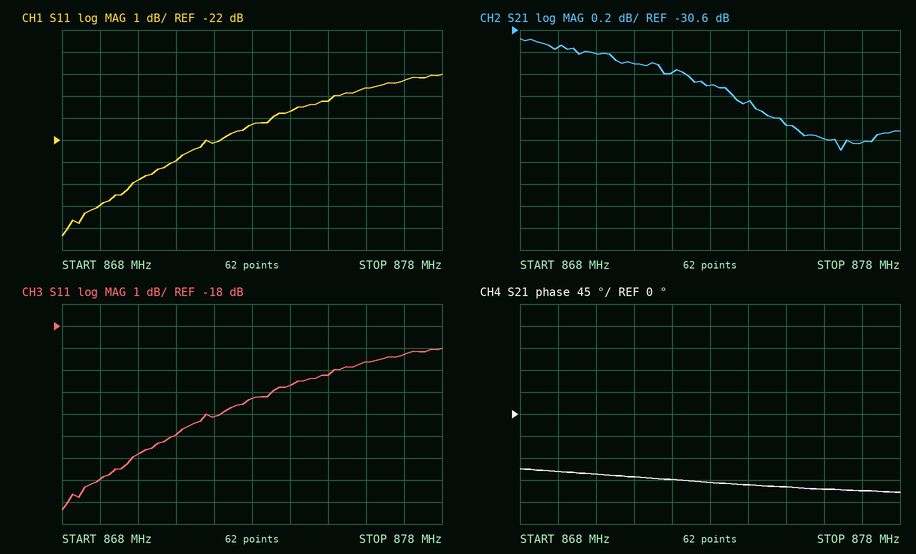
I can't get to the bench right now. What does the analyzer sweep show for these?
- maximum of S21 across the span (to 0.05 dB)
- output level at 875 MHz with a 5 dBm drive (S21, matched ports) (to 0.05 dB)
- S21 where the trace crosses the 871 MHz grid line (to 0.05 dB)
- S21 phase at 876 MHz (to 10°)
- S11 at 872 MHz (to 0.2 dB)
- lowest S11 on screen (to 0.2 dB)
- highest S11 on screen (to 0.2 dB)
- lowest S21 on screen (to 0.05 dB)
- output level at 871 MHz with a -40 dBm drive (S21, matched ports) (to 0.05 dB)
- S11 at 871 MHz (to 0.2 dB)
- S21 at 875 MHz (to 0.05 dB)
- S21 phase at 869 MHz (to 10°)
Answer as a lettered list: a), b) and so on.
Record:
a) -30.70 dB
b) -26.45 dBm
c) -30.90 dB
d) -150°
e) -22.2 dB
f) -26.4 dB
g) -19.0 dB
h) -31.70 dB
i) -70.90 dBm
j) -23.0 dB
k) -31.45 dB
l) -120°
